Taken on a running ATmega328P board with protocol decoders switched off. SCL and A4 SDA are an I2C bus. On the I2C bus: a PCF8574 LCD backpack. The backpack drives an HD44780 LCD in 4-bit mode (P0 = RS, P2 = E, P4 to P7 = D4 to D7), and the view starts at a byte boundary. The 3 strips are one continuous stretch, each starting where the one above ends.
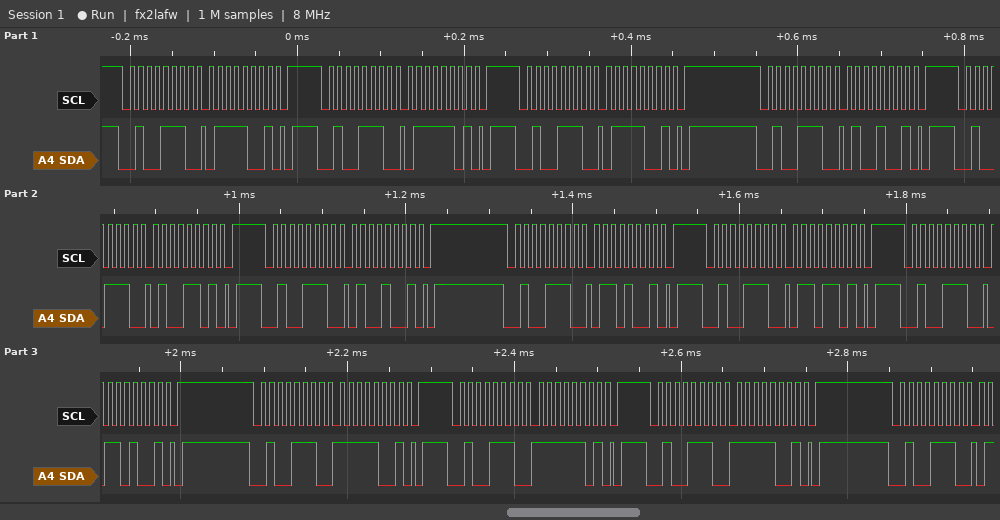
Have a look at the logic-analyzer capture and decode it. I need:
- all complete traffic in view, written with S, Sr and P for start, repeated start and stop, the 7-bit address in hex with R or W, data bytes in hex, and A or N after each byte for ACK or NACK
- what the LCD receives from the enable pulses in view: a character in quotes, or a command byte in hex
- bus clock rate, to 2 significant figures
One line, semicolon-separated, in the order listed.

S 27W A 79 A P S 27W A 7D A P S 27W A 79 A P S 27W A 49 A P S 27W A 4D A P S 27W A 49 A P S 27W A 69 A P S 27W A 6D A P S 27W A 69 A P S 27W A F9 A P S 27W A FD A P S 27W A F9 A P S 27W A; 't' 'o'; 100 kHz
